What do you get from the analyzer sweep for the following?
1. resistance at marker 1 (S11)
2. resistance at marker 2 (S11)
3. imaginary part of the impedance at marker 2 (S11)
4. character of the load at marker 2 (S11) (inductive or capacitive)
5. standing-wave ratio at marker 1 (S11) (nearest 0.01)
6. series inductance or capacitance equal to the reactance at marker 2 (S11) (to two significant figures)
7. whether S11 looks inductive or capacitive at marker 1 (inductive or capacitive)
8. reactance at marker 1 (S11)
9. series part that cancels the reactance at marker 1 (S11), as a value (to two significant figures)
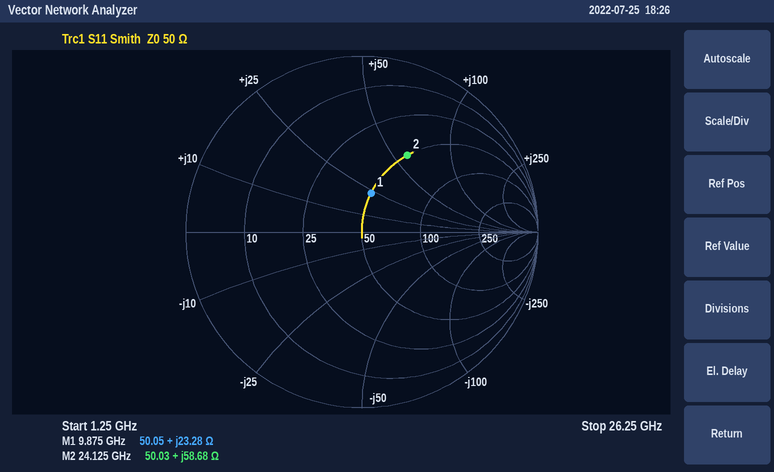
50.05 Ω
50.03 Ω
+58.68 Ω
inductive
1.59
390 pH
inductive
+23.28 Ω
690 fF
